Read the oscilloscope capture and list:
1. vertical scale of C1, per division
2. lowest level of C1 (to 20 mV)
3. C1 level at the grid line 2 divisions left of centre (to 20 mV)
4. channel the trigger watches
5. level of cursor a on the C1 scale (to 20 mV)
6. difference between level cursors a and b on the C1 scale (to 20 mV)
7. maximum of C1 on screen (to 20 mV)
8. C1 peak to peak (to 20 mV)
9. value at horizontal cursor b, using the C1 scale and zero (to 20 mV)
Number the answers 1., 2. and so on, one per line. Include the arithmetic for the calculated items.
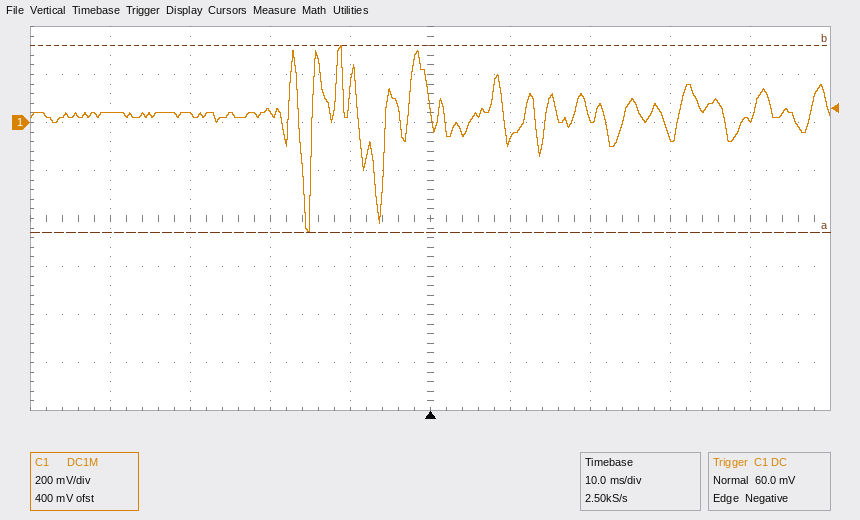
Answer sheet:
1. 200 mV
2. -460 mV
3. 40 mV
4. C1
5. -460 mV
6. 780 mV
7. 320 mV
8. 320 mV − (-460 mV) = 780 mV
9. 320 mV
